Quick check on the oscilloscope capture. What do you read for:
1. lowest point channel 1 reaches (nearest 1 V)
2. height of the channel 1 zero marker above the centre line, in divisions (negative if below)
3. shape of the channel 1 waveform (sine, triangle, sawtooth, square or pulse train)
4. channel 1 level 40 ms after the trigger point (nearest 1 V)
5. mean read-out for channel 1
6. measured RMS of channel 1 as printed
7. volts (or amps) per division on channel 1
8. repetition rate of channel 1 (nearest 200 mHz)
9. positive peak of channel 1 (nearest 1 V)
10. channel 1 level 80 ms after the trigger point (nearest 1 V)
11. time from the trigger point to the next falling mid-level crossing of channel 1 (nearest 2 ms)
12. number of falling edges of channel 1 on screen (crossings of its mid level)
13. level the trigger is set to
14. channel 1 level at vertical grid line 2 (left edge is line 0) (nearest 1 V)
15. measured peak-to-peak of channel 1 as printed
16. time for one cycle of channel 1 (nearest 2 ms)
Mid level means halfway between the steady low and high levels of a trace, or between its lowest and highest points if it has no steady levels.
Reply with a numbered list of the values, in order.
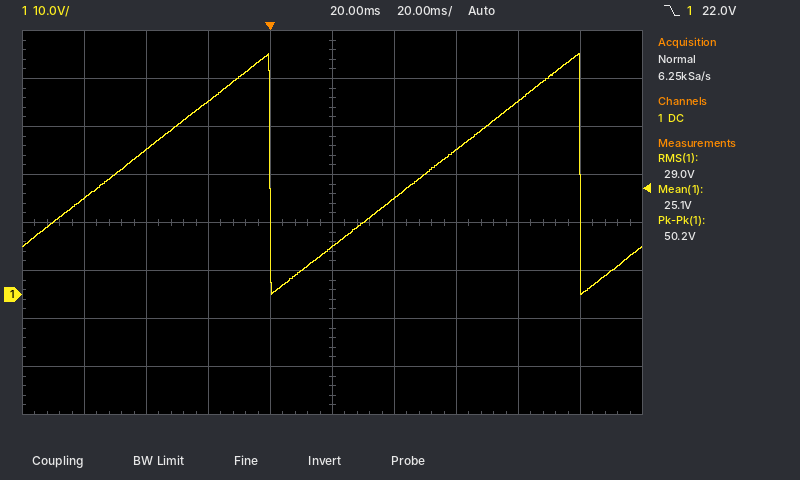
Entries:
1. 0 V
2. -1.5 div
3. sawtooth
4. 20 V
5. 25.1 V
6. 29.0 V
7. 10 V
8. 10.0 Hz
9. 50 V
10. 40 V
11. 100 ms
12. 2
13. 22.0 V
14. 30 V
15. 50.2 V
16. 100 ms
